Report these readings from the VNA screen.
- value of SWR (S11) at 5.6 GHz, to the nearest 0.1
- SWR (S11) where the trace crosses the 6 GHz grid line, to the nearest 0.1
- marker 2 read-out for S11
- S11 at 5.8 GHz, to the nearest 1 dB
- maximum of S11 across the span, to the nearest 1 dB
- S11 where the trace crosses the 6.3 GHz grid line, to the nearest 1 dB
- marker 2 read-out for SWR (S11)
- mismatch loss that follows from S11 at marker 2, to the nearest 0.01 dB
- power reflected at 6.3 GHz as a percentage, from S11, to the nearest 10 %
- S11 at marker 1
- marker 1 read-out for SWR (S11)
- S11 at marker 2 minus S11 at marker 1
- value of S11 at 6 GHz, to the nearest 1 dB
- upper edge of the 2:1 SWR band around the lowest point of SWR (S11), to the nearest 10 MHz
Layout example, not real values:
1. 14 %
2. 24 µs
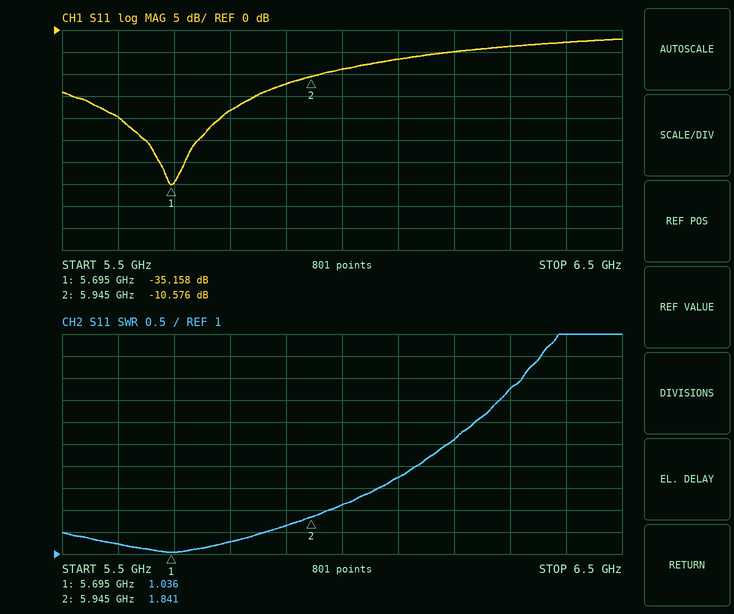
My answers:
1. 1.2
2. 2.1
3. -10.576 dB
4. -18 dB
5. -2 dB
6. -4 dB
7. 1.841
8. 0.40 dB
9. 40 %
10. -35.158 dB
11. 1.036
12. 24.582 dB
13. -9 dB
14. 5.98 GHz
